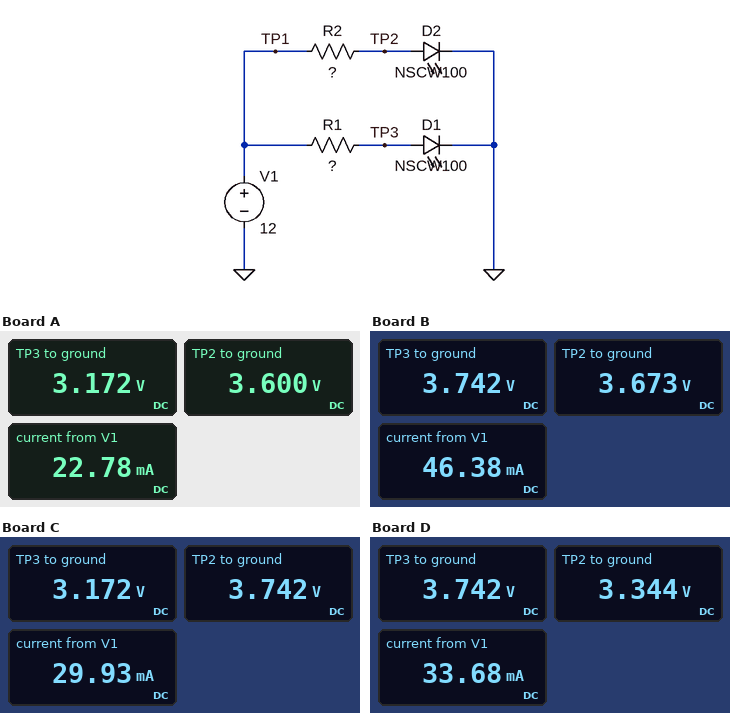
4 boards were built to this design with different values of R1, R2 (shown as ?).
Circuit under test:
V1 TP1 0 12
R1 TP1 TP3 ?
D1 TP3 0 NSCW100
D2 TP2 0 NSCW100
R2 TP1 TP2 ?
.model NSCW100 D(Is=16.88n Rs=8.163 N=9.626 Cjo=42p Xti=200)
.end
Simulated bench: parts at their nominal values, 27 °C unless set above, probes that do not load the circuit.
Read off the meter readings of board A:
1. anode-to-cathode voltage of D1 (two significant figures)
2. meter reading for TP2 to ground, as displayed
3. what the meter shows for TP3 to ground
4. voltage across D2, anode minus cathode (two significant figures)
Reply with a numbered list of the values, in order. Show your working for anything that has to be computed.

1. 3.172 V = 3.2 V
2. 3.600 V
3. 3.172 V
4. 3.6 V = 3.6 V
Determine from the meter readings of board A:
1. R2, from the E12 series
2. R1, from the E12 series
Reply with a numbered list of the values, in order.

1. 470 Ω
2. 1.8 kΩ
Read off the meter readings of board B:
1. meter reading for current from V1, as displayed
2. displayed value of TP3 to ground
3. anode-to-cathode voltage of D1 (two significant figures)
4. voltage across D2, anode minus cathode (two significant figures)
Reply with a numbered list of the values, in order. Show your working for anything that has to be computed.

1. 46.38 mA
2. 3.742 V
3. 3.742 V = 3.7 V
4. 3.673 V = 3.7 V
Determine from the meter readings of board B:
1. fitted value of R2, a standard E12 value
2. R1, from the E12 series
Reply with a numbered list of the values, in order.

1. 390 Ω
2. 330 Ω
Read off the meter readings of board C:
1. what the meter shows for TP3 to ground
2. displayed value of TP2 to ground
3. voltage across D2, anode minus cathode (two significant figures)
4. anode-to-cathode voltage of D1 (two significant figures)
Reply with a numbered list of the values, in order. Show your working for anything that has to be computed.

1. 3.172 V
2. 3.742 V
3. 3.742 V = 3.7 V
4. 3.172 V = 3.2 V
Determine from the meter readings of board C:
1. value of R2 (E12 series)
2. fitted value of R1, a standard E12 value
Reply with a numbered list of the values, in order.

1. 330 Ω
2. 1.8 kΩ
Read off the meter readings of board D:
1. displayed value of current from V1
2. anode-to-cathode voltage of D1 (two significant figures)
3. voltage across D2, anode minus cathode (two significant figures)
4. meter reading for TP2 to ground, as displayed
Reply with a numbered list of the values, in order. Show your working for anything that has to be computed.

1. 33.68 mA
2. 3.742 V = 3.7 V
3. 3.344 V = 3.3 V
4. 3.344 V
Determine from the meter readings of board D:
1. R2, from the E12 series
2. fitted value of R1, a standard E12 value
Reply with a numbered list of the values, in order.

1. 1 kΩ
2. 330 Ω
